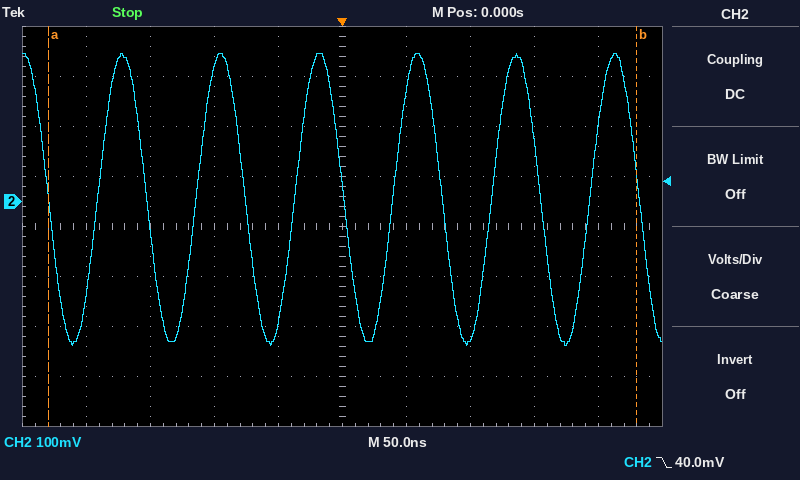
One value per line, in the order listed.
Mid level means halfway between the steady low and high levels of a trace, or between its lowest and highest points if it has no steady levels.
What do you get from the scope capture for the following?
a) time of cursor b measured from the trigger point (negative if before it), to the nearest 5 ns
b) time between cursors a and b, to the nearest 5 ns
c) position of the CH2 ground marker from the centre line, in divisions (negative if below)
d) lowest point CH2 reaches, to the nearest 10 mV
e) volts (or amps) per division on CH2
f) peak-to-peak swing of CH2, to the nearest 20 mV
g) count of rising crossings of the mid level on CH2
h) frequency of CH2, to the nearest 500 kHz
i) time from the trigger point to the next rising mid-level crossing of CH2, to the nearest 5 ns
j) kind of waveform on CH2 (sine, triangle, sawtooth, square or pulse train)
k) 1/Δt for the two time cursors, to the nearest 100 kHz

+230 ns
460 ns
+0.5 div
-290 mV
100 mV
580 mV
6
13.0 MHz
40 ns
sine
2.2 MHz
